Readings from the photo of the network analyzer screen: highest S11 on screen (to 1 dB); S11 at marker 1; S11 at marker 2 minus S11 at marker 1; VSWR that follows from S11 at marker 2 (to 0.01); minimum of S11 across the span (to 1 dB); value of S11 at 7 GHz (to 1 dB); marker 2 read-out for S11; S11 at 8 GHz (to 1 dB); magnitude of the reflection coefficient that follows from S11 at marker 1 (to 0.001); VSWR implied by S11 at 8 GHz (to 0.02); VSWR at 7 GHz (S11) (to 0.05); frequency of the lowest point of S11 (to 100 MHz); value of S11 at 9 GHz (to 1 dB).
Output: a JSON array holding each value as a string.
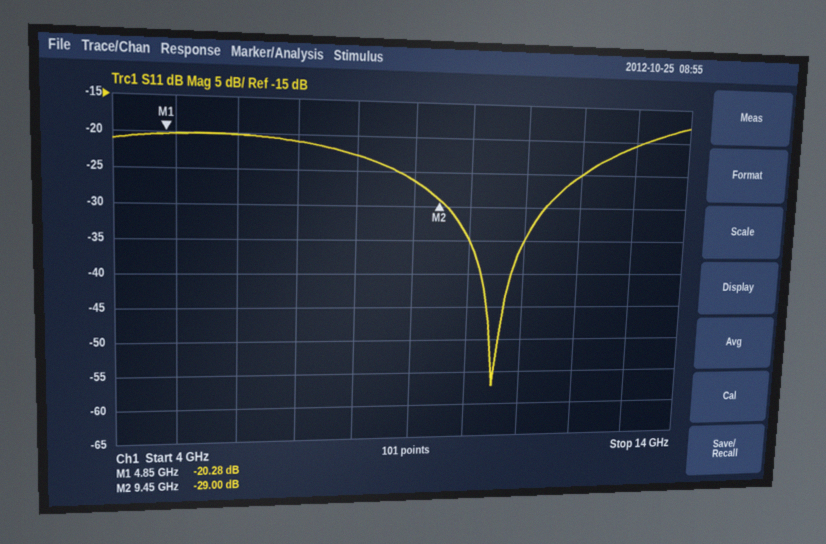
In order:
["-18 dB", "-20.28 dB", "-8.72 dB", "1.07", "-57 dB", "-21 dB", "-29.00 dB", "-23 dB", "0.097", "1.16", "1.20", "10.5 GHz", "-26 dB"]
